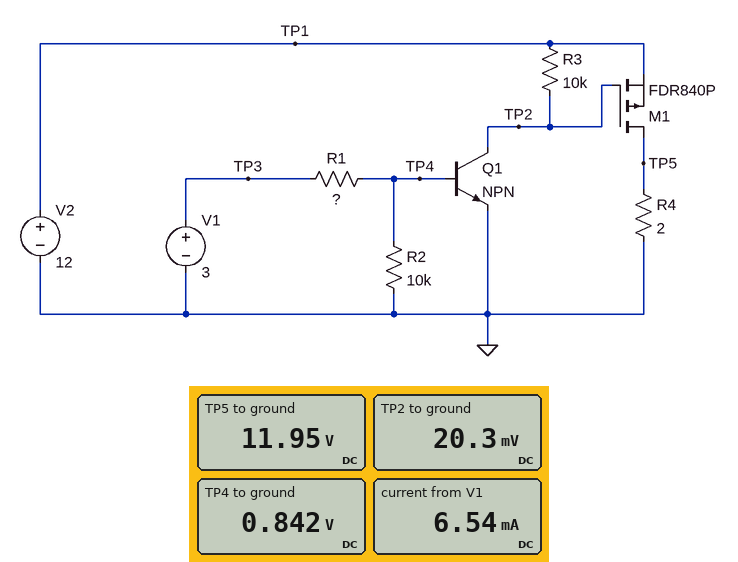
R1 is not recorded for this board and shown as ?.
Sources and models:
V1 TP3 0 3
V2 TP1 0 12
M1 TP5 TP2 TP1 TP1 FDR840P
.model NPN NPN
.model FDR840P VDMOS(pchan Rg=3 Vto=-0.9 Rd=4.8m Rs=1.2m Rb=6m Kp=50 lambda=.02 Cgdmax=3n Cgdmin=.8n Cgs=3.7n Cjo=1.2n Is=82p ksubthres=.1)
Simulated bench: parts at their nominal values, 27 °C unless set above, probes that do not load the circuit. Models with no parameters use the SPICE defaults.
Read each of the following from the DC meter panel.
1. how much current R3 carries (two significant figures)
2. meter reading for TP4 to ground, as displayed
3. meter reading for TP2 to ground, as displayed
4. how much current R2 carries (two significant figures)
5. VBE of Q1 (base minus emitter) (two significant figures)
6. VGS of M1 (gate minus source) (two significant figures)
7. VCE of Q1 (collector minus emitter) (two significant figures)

1.2 mA
0.842 V
20.3 mV
84 µA
840 mV
-12 V
20 mV
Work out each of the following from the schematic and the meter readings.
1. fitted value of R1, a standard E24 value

330 Ω
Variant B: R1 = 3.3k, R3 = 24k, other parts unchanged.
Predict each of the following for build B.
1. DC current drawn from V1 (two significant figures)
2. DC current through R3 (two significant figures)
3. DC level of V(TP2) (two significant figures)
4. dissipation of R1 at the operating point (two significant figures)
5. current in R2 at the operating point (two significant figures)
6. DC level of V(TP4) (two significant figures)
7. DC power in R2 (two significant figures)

670 µA
500 µA
27 mV
1.5 mW
79 µA
790 mV
62 µW
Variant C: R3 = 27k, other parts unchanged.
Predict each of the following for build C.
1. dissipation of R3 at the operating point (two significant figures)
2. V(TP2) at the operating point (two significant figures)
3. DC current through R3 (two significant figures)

5.3 mW
19 mV
440 µA
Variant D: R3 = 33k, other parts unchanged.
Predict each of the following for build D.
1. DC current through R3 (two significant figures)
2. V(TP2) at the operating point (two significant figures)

360 µA
19 mV
